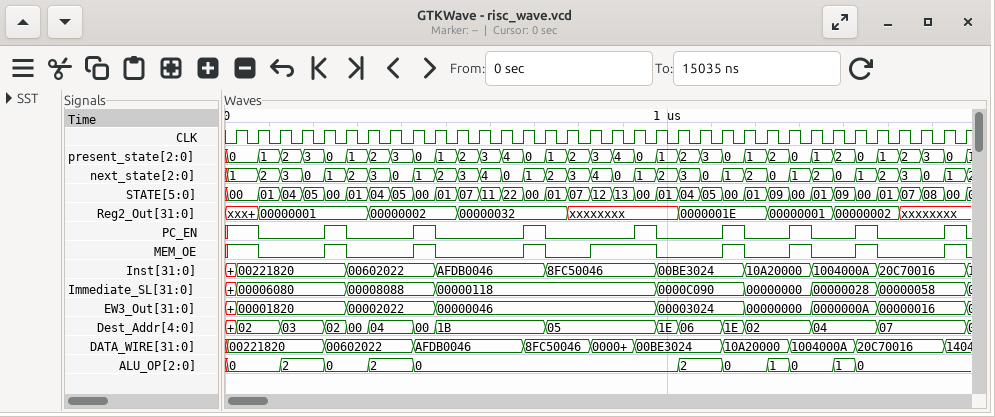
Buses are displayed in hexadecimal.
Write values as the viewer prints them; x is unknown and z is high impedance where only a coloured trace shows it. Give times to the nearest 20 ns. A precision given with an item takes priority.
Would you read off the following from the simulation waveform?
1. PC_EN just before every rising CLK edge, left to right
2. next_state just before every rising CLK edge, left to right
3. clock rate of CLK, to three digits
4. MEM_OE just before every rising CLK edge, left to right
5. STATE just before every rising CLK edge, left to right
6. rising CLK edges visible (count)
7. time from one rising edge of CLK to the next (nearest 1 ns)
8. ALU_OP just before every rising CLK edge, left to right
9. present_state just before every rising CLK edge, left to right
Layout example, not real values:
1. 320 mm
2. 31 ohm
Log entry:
1. 1 1 0 0 0 1 0 0 0 1 0 0 0 0 1 0 0 0 0 1 0 0 0 1 0 0 1 0 0 1 0 0 0 1
2. 1, 1, 2, 3, 0, 1, 2, 3, 0, 1, 2, 3, 4, 0, 1, 2, 3, 4, 0, 1, 2, 3, 0, 1, 2, 0, 1, 2, 0, 1, 2, 3, 0, 1
3. 20.0 MHz
4. 1 1 0 0 0 1 0 0 0 1 0 0 0 0 1 0 0 1 1 1 0 0 0 1 0 0 1 0 0 1 0 0 0 1
5. 00, 00, 01, 04, 05, 00, 01, 04, 05, 00, 01, 07, 11, 22, 00, 01, 07, 12, 13, 00, 01, 04, 05, 00, 01, 09, 00, 01, 09, 00, 01, 07, 08, 00
6. 34
7. 50 ns
8. 0, 0, 0, 2, 2, 0, 0, 2, 2, 0, 0, 0, 0, 0, 0, 0, 0, 0, 0, 0, 0, 2, 2, 0, 0, 1, 0, 0, 1, 0, 0, 0, 0, 0
9. 0, 0, 1, 2, 3, 0, 1, 2, 3, 0, 1, 2, 3, 4, 0, 1, 2, 3, 4, 0, 1, 2, 3, 0, 1, 2, 0, 1, 2, 0, 1, 2, 3, 0
